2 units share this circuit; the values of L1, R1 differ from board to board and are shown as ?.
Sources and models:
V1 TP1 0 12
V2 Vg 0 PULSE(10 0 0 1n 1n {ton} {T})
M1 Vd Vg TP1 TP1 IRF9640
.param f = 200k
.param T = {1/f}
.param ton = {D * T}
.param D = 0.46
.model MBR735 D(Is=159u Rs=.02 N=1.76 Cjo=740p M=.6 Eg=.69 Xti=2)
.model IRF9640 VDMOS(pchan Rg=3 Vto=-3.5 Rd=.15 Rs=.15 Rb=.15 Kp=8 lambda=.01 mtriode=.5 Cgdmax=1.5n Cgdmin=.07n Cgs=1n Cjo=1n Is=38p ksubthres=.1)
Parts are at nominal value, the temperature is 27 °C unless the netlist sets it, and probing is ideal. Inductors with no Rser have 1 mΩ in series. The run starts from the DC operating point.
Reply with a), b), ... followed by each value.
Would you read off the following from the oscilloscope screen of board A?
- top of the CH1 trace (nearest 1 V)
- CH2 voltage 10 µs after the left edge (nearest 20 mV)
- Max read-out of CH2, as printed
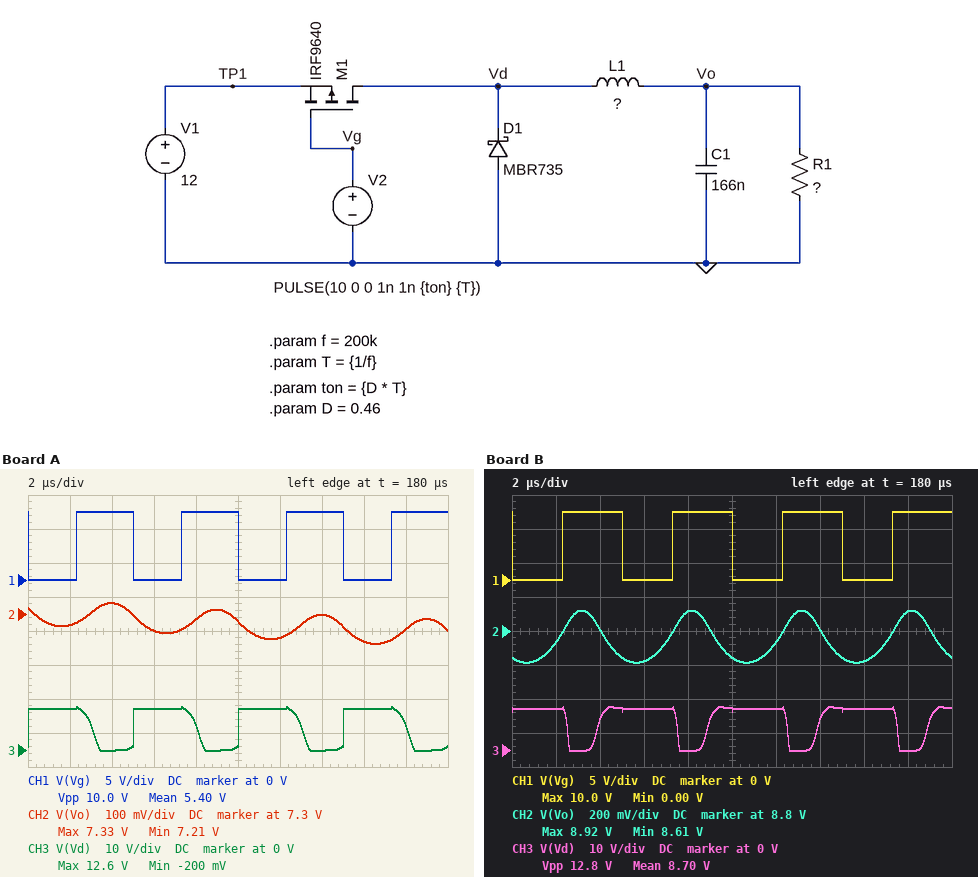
a) 10 V
b) 7.28 V
c) 7.33 V
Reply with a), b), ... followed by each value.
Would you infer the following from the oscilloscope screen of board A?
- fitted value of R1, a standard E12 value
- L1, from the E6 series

a) 1.2 kΩ
b) 680 µH
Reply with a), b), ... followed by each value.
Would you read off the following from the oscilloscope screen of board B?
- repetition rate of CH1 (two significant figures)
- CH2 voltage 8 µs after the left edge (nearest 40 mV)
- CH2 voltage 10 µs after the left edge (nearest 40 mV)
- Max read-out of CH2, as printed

a) 200 kHz
b) 8.92 V
c) 8.64 V
d) 8.92 V
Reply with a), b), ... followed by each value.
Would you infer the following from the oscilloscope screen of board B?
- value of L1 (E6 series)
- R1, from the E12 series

a) 150 µH
b) 560 Ω
